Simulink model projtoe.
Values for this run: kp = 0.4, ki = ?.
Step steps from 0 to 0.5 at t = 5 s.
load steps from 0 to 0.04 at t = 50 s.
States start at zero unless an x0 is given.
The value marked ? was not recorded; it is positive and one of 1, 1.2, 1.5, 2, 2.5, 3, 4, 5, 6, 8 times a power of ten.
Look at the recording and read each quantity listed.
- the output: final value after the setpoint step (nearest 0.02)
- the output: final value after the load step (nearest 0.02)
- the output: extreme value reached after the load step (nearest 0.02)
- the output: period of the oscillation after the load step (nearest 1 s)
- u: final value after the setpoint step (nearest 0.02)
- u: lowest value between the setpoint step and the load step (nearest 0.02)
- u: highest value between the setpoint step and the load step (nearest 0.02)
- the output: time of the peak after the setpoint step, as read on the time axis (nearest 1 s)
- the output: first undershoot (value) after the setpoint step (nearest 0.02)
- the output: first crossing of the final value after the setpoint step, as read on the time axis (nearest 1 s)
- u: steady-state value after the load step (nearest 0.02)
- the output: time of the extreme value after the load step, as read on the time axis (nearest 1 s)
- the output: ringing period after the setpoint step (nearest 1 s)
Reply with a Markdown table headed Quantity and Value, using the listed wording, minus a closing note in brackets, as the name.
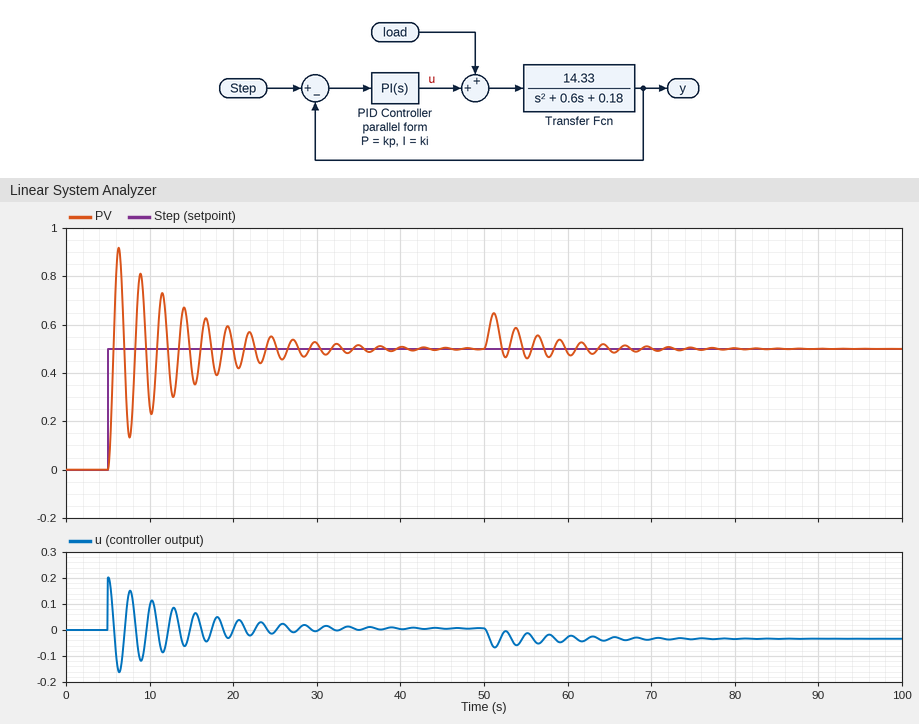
| Quantity | Value |
|---|---|
| the output: final value after the setpoint step | 0.50 |
| the output: final value after the load step | 0.50 |
| the output: extreme value reached after the load step | 0.64 |
| the output: period of the oscillation after the load step | 3 s |
| u: final value after the setpoint step | 0.00 |
| u: lowest value between the setpoint step and the load step | -0.16 |
| u: highest value between the setpoint step and the load step | 0.20 |
| the output: time of the peak after the setpoint step, as read on the time axis | 6 s |
| the output: first undershoot (value) after the setpoint step | 0.14 |
| the output: first crossing of the final value after the setpoint step, as read on the time axis | 6 s |
| u: steady-state value after the load step | -0.04 |
| the output: time of the extreme value after the load step, as read on the time axis | 51 s |
| the output: ringing period after the setpoint step | 3 s |
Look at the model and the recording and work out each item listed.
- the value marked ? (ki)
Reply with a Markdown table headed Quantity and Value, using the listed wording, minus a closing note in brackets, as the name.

| Quantity | Value |
|---|---|
| the value marked ? | 0.15 |
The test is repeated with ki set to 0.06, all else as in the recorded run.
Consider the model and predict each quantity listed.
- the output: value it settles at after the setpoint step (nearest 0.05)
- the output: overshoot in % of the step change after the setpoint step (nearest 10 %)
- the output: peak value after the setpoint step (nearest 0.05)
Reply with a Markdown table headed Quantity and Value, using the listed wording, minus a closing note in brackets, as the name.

| Quantity | Value |
|---|---|
| the output: value it settles at after the setpoint step | 0.50 |
| the output: overshoot in % of the step change after the setpoint step | 70 % |
| the output: peak value after the setpoint step | 0.85 |
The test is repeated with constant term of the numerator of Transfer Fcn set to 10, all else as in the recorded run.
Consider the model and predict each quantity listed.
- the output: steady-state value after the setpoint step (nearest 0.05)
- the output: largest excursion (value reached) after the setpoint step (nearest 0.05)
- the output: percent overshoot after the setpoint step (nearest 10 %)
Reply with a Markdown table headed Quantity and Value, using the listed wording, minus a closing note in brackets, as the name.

| Quantity | Value |
|---|---|
| the output: steady-state value after the setpoint step | 0.50 |
| the output: largest excursion (value reached) after the setpoint step | 0.90 |
| the output: percent overshoot after the setpoint step | 80 % |
